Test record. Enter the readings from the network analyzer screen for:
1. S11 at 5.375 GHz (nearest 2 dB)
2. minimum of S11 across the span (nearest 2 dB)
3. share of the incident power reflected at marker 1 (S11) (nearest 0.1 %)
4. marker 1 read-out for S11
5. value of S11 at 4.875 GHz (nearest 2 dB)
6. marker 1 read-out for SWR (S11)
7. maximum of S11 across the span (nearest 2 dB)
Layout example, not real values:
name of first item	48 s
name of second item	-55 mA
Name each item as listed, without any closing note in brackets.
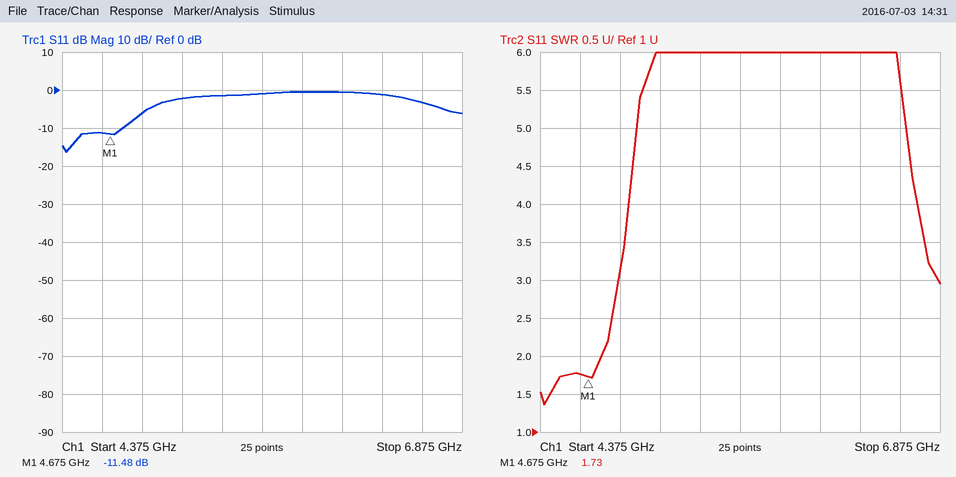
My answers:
S11 at 5.375 GHz	-2 dB
minimum of S11 across the span	-16 dB
share of the incident power reflected at marker 1 (S11)	7.1 %
marker 1 read-out for S11	-11.48 dB
value of S11 at 4.875 GHz	-6 dB
marker 1 read-out for SWR	1.73
maximum of S11 across the span	0 dB
